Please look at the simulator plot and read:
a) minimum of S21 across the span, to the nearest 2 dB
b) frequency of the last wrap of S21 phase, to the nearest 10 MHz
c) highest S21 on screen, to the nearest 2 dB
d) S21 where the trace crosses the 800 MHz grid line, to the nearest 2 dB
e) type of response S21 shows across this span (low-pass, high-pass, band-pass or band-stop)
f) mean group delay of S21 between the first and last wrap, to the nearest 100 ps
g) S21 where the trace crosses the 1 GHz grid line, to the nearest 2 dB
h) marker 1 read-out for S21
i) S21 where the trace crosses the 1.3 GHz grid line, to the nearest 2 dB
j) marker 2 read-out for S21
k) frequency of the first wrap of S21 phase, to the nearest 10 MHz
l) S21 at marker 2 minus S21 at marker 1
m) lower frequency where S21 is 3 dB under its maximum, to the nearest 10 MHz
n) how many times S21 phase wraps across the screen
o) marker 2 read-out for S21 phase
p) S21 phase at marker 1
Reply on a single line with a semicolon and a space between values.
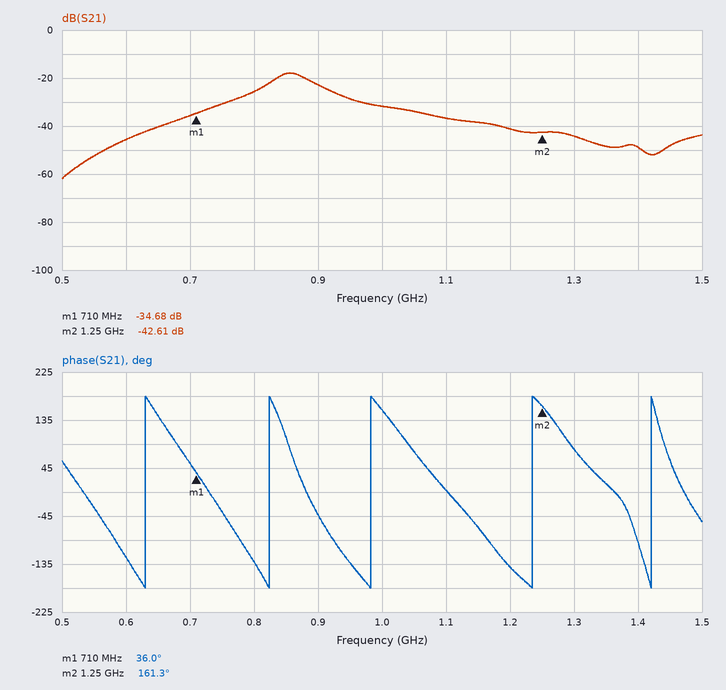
-62 dB; 1.42 GHz; -18 dB; -26 dB; band-pass; 5.1 ns; -32 dB; -34.68 dB; -44 dB; -42.61 dB; 630 MHz; -7.93 dB; 830 MHz; 5; 161.3°; 36.0°
